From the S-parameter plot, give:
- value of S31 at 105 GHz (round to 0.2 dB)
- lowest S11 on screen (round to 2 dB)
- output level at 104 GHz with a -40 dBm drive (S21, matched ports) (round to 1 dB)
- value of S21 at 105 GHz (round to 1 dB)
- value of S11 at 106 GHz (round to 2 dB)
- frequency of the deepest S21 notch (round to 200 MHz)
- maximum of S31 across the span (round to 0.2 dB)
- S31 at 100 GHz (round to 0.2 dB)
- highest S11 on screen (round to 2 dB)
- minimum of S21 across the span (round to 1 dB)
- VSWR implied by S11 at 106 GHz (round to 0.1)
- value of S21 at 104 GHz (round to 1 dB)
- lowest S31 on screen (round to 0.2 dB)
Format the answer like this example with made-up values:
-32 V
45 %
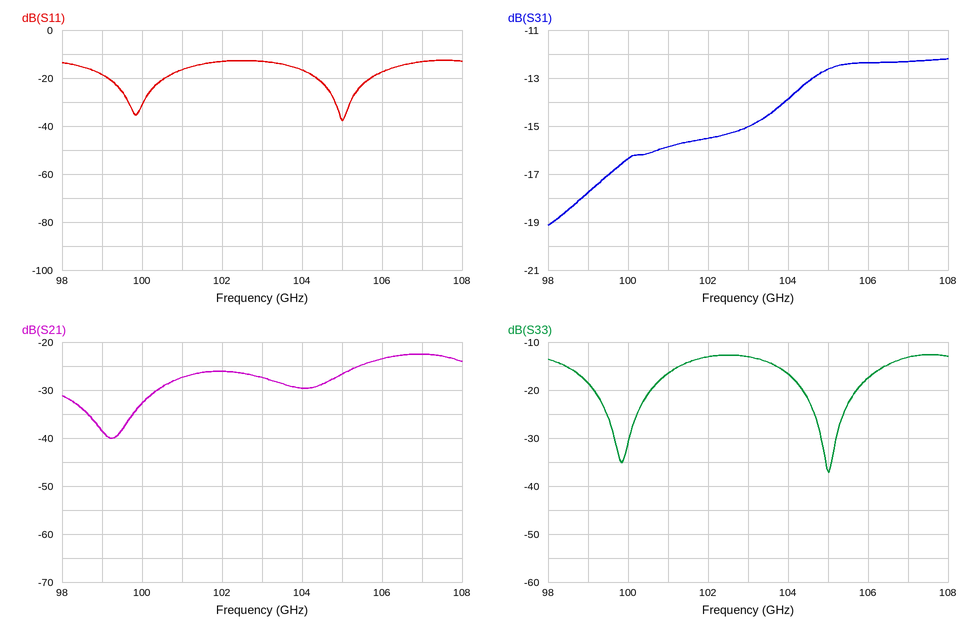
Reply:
-12.6 dB
-38 dB
-70 dBm
-27 dB
-18 dB
99.2 GHz
-12.2 dB
-16.4 dB
-12 dB
-40 dB
1.3
-30 dB
-19.2 dB
